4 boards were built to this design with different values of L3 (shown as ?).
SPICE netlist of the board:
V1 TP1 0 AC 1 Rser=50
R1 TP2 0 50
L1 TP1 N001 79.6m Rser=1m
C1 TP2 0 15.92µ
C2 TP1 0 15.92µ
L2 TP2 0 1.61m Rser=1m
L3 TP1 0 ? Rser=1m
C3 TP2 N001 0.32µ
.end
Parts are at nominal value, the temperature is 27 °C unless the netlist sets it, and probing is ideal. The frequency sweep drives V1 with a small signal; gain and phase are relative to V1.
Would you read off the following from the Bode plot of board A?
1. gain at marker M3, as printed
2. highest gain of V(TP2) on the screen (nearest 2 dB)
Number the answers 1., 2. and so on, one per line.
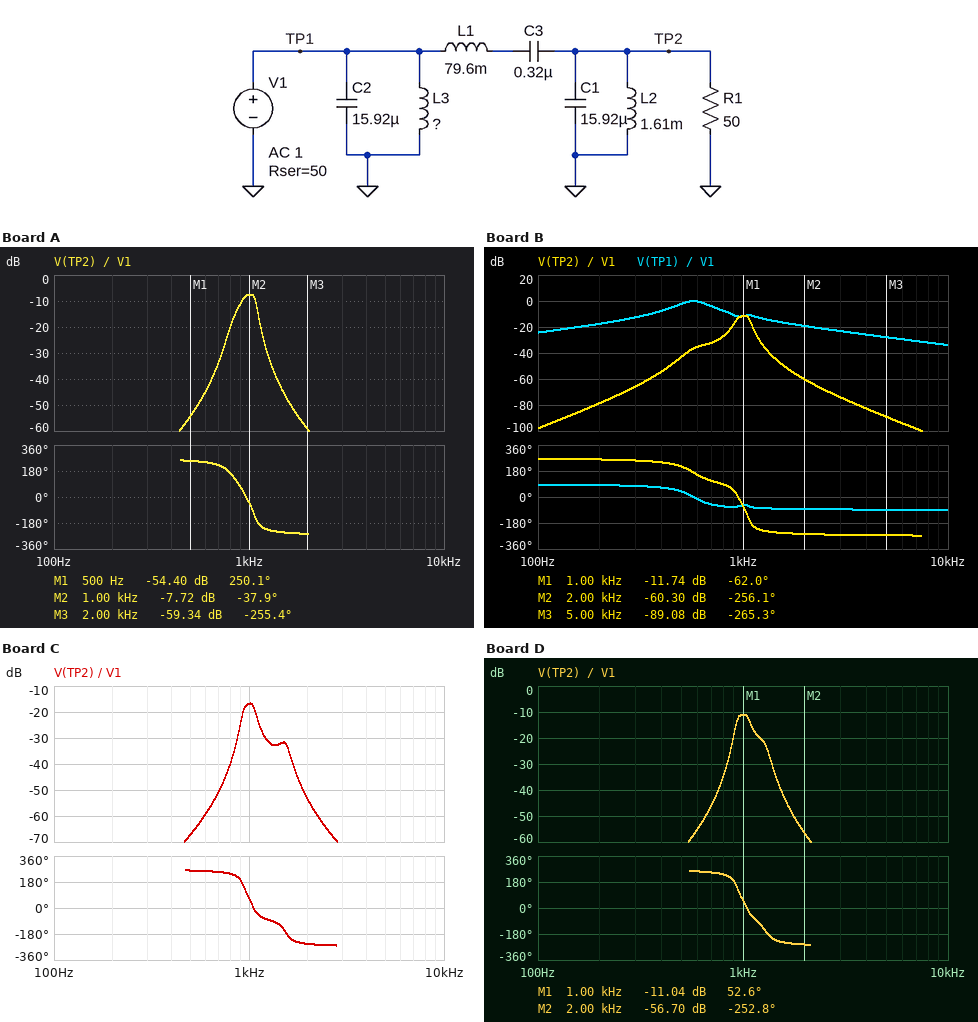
1. -59.34 dB
2. -8 dB
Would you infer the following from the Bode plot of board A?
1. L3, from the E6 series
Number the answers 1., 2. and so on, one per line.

1. 2.2 mH
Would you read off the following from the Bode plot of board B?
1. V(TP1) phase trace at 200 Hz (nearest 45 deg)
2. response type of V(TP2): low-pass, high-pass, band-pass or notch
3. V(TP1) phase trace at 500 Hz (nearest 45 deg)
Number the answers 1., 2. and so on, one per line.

1. 90 deg
2. band-pass
3. 45 deg
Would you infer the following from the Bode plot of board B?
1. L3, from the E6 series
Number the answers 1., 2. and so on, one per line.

1. 4.7 mH
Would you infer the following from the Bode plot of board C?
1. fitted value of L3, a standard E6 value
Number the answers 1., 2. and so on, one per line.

1. 680 µH
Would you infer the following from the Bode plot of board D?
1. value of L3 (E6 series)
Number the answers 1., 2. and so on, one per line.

1. 1 mH
